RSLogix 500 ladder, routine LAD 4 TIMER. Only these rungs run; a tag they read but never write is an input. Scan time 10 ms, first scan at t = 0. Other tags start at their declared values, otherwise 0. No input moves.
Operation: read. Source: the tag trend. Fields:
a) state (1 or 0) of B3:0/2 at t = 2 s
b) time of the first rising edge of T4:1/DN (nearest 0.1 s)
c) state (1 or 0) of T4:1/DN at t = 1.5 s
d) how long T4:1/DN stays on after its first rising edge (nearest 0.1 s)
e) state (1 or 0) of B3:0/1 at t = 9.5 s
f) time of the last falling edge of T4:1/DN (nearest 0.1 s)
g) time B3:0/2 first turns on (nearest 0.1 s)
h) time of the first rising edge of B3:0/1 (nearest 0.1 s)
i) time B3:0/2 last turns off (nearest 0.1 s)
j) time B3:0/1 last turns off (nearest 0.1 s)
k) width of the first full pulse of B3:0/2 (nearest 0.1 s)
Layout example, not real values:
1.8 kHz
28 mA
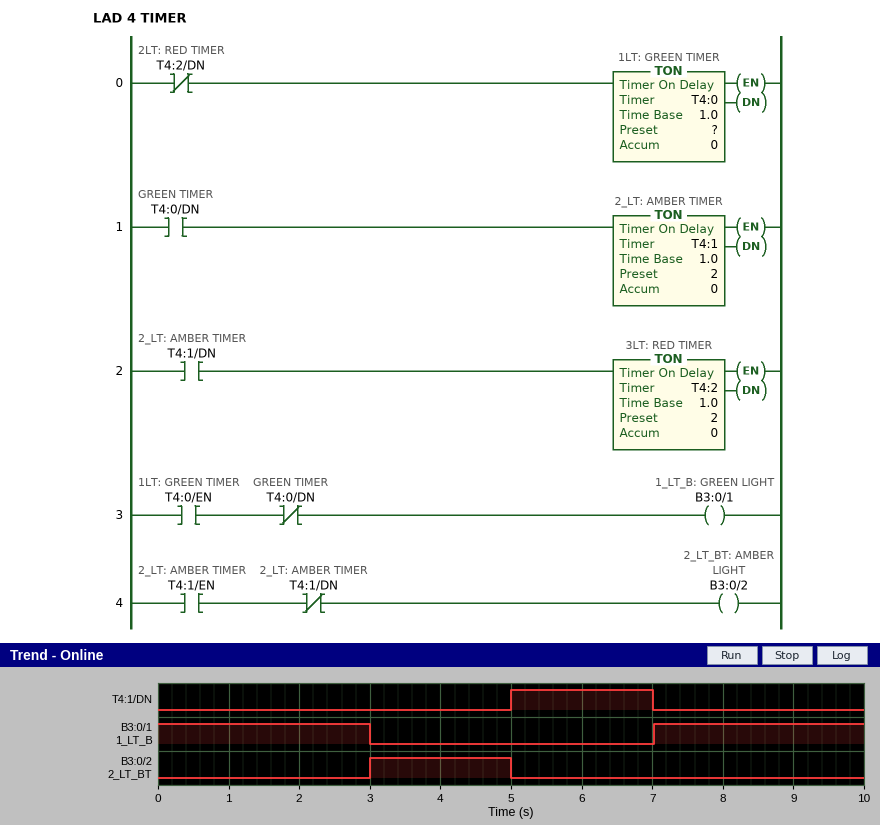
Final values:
0
5.0 s
0
2.0 s
1
7.0 s
3.0 s
7.0 s
5.0 s
3.0 s
2.0 s
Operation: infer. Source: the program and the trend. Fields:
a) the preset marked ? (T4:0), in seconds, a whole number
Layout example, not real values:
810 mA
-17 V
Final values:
3 s
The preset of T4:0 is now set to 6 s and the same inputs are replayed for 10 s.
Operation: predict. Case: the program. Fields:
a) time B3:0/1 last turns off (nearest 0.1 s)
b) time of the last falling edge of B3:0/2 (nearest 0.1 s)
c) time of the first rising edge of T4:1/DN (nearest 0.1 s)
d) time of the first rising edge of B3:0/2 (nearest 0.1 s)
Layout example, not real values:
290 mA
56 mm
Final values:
6.0 s
8.0 s
8.0 s
6.0 s
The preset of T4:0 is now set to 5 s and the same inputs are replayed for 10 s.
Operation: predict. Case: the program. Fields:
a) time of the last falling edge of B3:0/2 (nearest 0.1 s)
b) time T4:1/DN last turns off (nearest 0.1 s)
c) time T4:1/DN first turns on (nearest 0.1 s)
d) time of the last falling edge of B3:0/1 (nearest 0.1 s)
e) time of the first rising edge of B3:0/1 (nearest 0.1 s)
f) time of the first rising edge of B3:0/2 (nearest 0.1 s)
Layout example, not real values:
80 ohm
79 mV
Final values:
7.0 s
9.0 s
7.0 s
5.0 s
9.0 s
5.0 s
